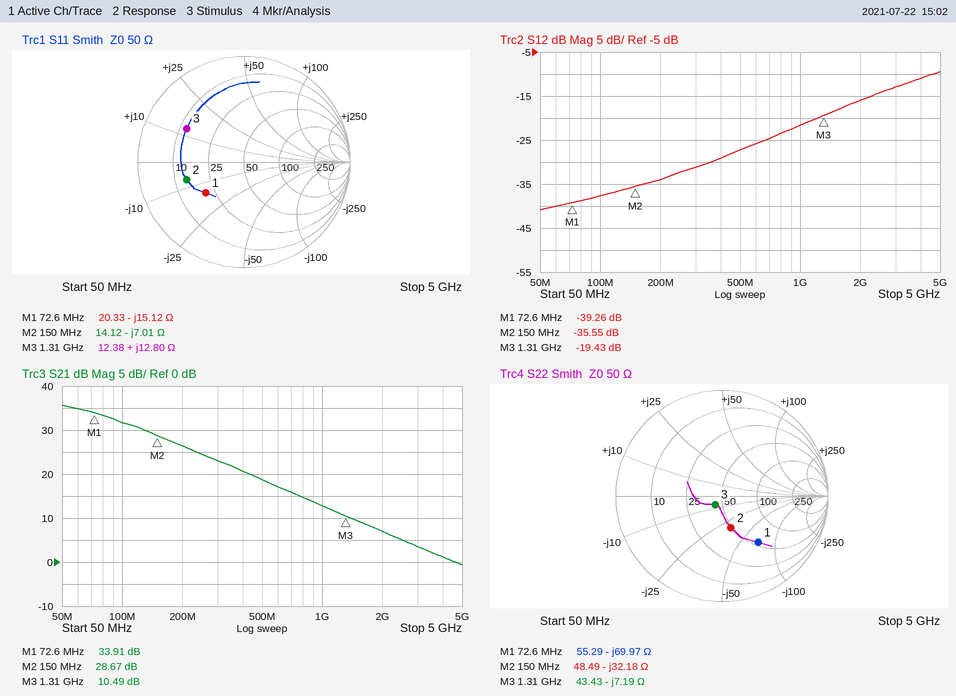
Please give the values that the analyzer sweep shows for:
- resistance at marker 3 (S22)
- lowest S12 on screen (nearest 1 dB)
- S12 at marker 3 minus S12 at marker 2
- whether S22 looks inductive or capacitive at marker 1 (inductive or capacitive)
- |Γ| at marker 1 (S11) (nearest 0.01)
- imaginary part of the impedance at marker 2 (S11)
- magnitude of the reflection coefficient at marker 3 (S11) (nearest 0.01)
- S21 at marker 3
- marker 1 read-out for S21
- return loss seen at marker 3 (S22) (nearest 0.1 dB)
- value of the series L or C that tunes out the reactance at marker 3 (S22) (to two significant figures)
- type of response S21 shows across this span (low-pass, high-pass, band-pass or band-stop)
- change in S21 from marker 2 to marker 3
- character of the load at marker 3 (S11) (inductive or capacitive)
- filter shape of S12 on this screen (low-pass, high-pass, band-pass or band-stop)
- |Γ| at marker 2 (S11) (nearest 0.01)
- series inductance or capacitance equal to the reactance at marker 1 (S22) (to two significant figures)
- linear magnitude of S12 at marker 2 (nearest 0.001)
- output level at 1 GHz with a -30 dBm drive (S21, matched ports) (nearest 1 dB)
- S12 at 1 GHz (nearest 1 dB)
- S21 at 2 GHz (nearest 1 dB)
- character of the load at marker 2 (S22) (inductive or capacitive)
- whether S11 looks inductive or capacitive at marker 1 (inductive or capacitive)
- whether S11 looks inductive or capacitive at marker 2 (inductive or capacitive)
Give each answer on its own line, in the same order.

43.43 Ω
-41 dB
16.12 dB
capacitive
0.46
-7.01 Ω
0.62
10.49 dB
33.91 dB
19.7 dB
870 pH
low-pass
-18.18 dB
inductive
high-pass
0.57
31 pF
0.017
-17 dBm
-22 dB
7 dB
capacitive
capacitive
capacitive
